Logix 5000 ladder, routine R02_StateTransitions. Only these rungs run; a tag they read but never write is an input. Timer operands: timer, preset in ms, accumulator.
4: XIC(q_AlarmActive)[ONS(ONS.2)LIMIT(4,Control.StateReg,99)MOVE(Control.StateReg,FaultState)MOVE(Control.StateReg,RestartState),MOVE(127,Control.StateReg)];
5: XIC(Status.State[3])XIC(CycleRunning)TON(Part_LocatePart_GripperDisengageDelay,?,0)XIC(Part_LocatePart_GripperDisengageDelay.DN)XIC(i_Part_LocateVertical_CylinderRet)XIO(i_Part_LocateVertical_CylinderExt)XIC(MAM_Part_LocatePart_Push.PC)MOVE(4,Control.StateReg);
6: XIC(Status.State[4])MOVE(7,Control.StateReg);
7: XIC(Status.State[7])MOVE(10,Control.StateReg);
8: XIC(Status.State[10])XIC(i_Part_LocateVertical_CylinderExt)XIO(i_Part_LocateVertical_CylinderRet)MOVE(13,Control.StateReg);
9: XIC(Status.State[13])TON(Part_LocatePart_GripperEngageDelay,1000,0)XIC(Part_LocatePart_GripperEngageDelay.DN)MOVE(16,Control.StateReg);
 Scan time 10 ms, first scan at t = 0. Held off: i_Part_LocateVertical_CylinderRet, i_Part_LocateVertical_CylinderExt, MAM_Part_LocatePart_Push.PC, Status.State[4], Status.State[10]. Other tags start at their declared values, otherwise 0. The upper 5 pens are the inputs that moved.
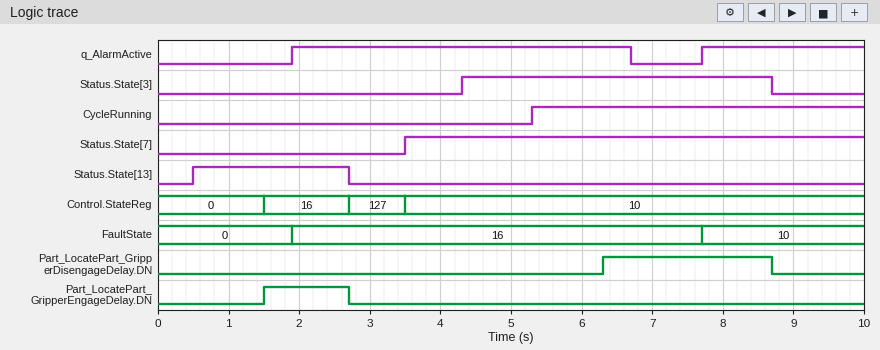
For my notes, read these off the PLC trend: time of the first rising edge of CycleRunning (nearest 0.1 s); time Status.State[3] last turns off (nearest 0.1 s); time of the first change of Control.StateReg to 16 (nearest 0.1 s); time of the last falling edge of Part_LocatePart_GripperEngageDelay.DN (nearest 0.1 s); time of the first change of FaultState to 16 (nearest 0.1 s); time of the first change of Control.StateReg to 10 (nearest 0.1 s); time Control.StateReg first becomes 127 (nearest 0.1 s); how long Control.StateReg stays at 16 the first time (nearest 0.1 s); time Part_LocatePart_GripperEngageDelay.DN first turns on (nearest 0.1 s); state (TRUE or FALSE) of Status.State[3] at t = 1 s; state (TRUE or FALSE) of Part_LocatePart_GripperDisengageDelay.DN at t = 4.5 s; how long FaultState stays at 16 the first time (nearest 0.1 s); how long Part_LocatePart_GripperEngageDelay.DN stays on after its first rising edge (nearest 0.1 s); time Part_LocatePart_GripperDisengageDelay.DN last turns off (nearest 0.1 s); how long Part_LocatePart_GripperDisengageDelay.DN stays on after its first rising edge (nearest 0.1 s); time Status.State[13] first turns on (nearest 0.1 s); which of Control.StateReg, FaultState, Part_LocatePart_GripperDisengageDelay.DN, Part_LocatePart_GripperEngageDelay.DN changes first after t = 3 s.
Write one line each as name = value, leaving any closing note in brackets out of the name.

time of the first rising edge of CycleRunning = 5.3 s
time Status.State[3] last turns off = 8.7 s
time of the first change of Control.StateReg to 16 = 1.5 s
time of the last falling edge of Part_LocatePart_GripperEngageDelay.DN = 2.7 s
time of the first change of FaultState to 16 = 1.9 s
time of the first change of Control.StateReg to 10 = 3.5 s
time Control.StateReg first becomes 127 = 2.7 s
how long Control.StateReg stays at 16 the first time = 1.2 s
time Part_LocatePart_GripperEngageDelay.DN first turns on = 1.5 s
state (TRUE or FALSE) of Status.State[3] at t = 1 s = FALSE
state (TRUE or FALSE) of Part_LocatePart_GripperDisengageDelay.DN at t = 4.5 s = FALSE
how long FaultState stays at 16 the first time = 5.8 s
how long Part_LocatePart_GripperEngageDelay.DN stays on after its first rising edge = 1.2 s
time Part_LocatePart_GripperDisengageDelay.DN last turns off = 8.7 s
how long Part_LocatePart_GripperDisengageDelay.DN stays on after its first rising edge = 2.4 s
time Status.State[13] first turns on = 0.5 s
which of Control.StateReg, FaultState, Part_LocatePart_GripperDisengageDelay.DN, Part_LocatePart_GripperEngageDelay.DN changes first after t = 3 s = Control.StateReg
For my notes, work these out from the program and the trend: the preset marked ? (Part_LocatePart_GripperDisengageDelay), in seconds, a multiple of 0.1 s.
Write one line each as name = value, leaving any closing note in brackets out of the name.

the preset marked ? (Part_LocatePart_GripperDisengageDelay), in seconds, a multiple of 0.1 s = 1.0 s
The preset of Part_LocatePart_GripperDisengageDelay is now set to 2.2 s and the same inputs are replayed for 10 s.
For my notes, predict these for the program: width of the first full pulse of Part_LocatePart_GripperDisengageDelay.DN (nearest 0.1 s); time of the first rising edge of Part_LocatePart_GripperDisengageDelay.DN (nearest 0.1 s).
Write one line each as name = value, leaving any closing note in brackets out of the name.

width of the first full pulse of Part_LocatePart_GripperDisengageDelay.DN = 1.2 s
time of the first rising edge of Part_LocatePart_GripperDisengageDelay.DN = 7.5 s
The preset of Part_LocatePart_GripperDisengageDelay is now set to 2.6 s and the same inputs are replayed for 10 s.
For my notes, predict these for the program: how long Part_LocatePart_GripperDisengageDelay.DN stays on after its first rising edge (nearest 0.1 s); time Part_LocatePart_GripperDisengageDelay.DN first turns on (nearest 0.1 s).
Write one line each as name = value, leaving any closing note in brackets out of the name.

how long Part_LocatePart_GripperDisengageDelay.DN stays on after its first rising edge = 0.8 s
time Part_LocatePart_GripperDisengageDelay.DN first turns on = 7.9 s
